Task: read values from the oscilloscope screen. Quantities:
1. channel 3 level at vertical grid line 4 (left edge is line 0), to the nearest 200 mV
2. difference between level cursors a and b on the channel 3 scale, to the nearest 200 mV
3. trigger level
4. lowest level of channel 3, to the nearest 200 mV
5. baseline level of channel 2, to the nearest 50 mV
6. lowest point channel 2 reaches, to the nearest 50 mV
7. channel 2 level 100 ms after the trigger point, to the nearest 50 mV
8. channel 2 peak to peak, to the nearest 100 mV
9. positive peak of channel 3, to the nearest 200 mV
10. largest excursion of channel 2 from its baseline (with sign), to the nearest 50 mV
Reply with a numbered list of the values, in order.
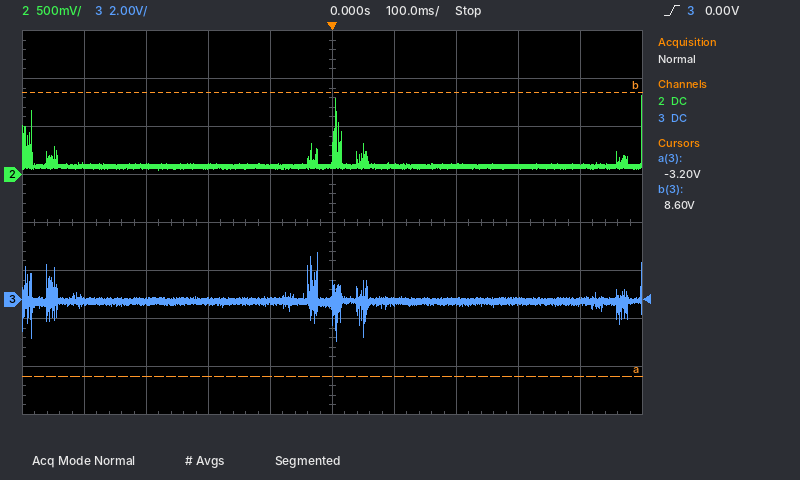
1. 0.0 V
2. 11.8 V
3. 0.00 V
4. -1.8 V
5. 100 mV
6. 50 mV
7. 100 mV
8. 800 mV
9. 2.0 V
10. +750 mV
